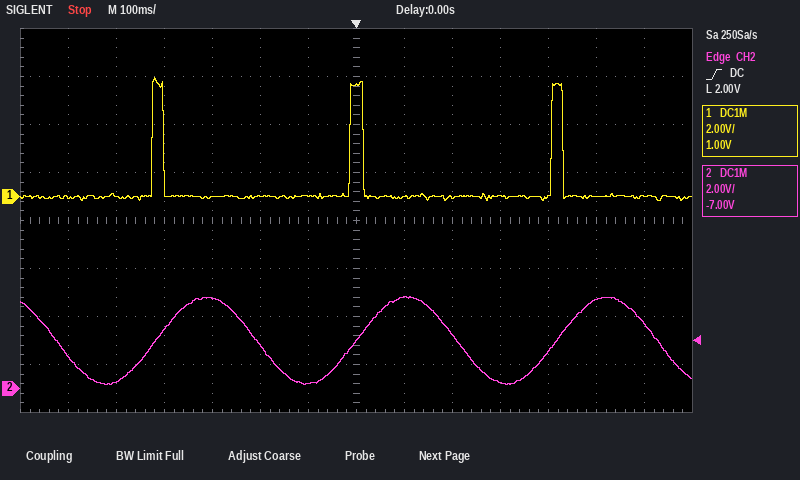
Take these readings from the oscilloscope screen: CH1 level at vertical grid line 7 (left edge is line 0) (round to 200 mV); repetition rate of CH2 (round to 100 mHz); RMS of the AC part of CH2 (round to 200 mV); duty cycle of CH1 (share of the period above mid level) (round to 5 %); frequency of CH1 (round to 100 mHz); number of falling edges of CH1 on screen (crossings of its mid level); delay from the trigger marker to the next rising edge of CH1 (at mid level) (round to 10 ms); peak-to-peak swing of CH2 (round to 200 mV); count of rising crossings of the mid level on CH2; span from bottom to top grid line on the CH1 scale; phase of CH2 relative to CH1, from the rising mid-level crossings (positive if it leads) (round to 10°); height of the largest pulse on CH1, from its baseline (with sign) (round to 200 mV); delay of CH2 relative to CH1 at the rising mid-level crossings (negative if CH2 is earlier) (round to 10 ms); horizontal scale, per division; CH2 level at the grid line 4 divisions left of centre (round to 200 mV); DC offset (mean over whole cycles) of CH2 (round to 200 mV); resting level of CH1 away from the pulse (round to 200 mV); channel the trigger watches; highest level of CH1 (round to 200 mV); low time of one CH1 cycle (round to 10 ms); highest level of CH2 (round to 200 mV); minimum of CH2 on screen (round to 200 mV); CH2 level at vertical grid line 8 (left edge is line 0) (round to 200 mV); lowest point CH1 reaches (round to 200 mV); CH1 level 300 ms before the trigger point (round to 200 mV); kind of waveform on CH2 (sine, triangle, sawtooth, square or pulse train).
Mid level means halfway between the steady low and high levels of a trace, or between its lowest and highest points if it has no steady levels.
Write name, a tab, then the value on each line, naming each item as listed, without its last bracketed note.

CH1 level at vertical grid line 7 (left edge is line 0)	4.6 V
repetition rate of CH2	2.4 Hz
RMS of the AC part of CH2	1.2 V
duty cycle of CH1 (share of the period above mid level)	5 %
frequency of CH1	2.4 Hz
number of falling edges of CH1 on screen	3
delay from the trigger marker to the next rising edge of CH1 (at mid level)	410 ms
peak-to-peak swing of CH2	3.6 V
count of rising crossings of the mid level on CH2	3
span from bottom to top grid line on the CH1 scale	16 V
phase of CH2 relative to CH1, from the rising mid-level crossings (positive if it leads)	-10°
height of the largest pulse on CH1, from its baseline (with sign)	+5.0 V
delay of CH2 relative to CH1 at the rising mid-level crossings (negative if CH2 is earlier)	+10 ms
horizontal scale, per division	100 ms
CH2 level at the grid line 4 divisions left of centre	2.4 V
DC offset (mean over whole cycles) of CH2	2.0 V
resting level of CH1 away from the pulse	0.0 V
channel the trigger watches	CH2
highest level of CH1	5.0 V
low time of one CH1 cycle	390 ms
highest level of CH2	3.8 V
minimum of CH2 on screen	200 mV
CH2 level at vertical grid line 8 (left edge is line 0)	3.8 V
lowest point CH1 reaches	-200 mV
CH1 level 300 ms before the trigger point	0.0 V
kind of waveform on CH2	sine
